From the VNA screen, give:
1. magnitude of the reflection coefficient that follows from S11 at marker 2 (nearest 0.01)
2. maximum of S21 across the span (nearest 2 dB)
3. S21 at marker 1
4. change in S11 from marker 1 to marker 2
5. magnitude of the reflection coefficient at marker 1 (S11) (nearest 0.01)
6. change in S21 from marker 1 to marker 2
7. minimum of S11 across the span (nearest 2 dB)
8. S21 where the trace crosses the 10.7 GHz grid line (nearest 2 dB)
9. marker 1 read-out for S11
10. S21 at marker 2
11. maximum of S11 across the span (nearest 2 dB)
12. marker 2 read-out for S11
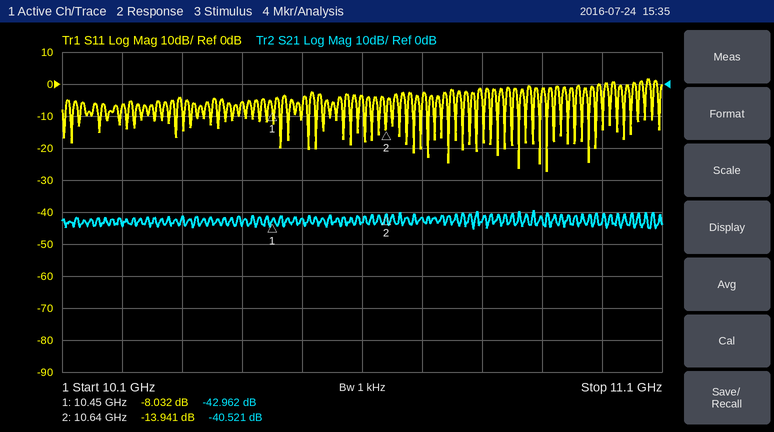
0.20
-40 dB
-42.962 dB
-5.909 dB
0.40
2.441 dB
-28 dB
-42 dB
-8.032 dB
-40.521 dB
2 dB
-13.941 dB
